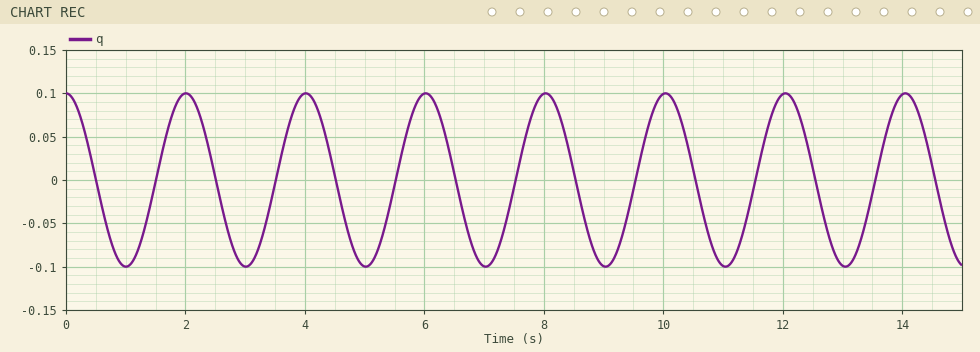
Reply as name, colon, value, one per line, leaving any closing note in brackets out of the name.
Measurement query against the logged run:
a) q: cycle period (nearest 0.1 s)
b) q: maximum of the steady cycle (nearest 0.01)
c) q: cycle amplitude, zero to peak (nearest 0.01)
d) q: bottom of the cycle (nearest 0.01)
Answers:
q: cycle period: 2.0 s
q: maximum of the steady cycle: 0.10
q: cycle amplitude, zero to peak: 0.10
q: bottom of the cycle: -0.10
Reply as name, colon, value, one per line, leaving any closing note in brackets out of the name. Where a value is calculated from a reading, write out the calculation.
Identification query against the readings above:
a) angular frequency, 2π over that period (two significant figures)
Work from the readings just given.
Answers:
angular frequency, 2π over that period: 2π / 2 = 3.1 rad/s
